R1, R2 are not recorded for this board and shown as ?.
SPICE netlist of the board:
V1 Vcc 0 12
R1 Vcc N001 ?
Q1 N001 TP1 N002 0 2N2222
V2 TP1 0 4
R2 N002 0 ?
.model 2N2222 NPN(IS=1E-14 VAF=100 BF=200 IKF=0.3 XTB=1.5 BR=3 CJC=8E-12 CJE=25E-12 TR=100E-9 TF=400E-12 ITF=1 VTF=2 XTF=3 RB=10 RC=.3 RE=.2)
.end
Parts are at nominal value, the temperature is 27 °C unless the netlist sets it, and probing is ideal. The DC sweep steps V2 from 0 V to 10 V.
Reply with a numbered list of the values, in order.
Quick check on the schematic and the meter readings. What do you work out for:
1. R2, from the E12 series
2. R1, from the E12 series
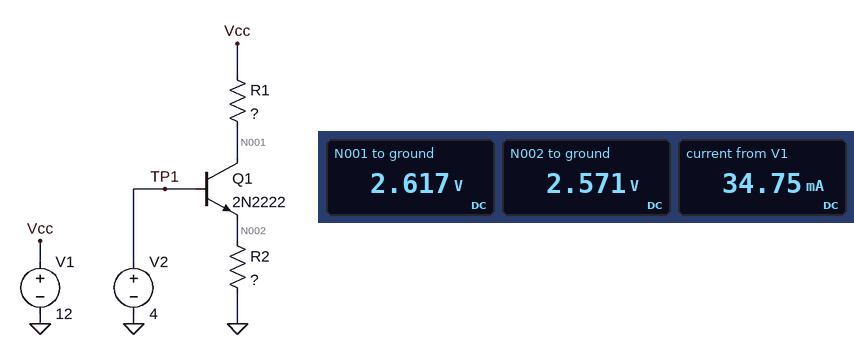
1. 27 Ω
2. 270 Ω
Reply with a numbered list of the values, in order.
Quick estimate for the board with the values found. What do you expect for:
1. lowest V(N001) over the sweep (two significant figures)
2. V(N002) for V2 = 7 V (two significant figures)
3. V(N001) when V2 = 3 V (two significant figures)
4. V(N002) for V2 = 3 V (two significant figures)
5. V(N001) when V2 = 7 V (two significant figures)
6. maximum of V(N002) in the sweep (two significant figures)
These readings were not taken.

1. 1.2 V
2. 4.7 V
3. 1.9 V
4. 1.9 V
5. 4.7 V
6. 6.8 V
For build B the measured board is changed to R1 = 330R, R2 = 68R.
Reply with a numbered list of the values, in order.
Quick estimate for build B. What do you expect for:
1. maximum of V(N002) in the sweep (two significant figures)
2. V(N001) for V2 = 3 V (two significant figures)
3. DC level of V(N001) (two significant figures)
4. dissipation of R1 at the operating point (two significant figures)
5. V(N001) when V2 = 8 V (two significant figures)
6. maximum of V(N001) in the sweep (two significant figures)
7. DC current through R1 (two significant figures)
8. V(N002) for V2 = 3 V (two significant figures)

1. 8.1 V
2. 2.3 V
3. 3.1 V
4. 240 mW
5. 6.4 V
6. 12 V
7. 27 mA
8. 2.2 V
